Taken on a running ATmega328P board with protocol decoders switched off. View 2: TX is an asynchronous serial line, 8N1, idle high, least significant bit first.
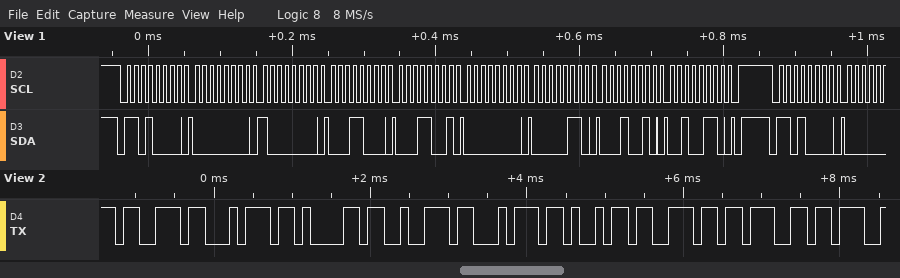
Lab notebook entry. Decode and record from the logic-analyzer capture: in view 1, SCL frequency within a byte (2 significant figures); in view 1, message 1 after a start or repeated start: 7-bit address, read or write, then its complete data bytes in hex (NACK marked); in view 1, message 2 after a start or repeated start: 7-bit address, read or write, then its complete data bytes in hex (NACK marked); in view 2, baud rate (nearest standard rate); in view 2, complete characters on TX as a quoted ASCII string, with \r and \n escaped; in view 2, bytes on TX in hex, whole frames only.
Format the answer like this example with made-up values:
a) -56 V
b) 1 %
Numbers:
a) 100 kHz
b) 0x68 write: 00 80 18 19 00 06 12 26
c) 0x68 write
d) 9600 baud
e) "starting"
f) 73 74 61 72 74 69 6E 67
